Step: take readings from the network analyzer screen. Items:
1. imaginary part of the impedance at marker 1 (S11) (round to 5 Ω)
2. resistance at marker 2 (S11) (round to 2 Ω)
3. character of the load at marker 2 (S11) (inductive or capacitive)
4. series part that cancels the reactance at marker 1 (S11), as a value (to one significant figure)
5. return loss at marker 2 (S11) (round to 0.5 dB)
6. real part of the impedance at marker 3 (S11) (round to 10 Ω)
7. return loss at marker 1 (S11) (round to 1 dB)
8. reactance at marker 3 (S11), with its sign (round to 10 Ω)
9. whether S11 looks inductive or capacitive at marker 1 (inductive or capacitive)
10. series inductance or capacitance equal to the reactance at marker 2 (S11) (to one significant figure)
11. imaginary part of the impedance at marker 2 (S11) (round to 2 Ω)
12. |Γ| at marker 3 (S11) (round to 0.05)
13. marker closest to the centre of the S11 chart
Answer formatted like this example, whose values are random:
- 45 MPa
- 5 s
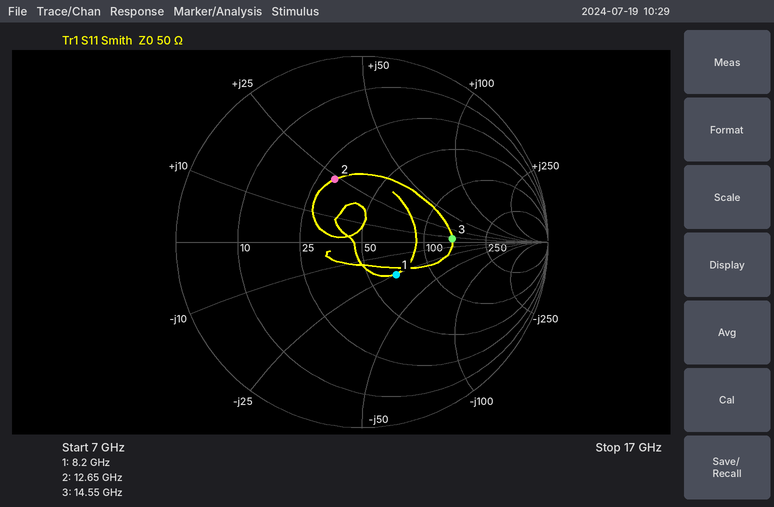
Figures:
- -25 Ω
- 30 Ω
- inductive
- 500 pH
- 8.5 dB
- 140 Ω
- 12 dB
- +10 Ω
- capacitive
- 300 pH
- +24 Ω
- 0.50
- marker 1
